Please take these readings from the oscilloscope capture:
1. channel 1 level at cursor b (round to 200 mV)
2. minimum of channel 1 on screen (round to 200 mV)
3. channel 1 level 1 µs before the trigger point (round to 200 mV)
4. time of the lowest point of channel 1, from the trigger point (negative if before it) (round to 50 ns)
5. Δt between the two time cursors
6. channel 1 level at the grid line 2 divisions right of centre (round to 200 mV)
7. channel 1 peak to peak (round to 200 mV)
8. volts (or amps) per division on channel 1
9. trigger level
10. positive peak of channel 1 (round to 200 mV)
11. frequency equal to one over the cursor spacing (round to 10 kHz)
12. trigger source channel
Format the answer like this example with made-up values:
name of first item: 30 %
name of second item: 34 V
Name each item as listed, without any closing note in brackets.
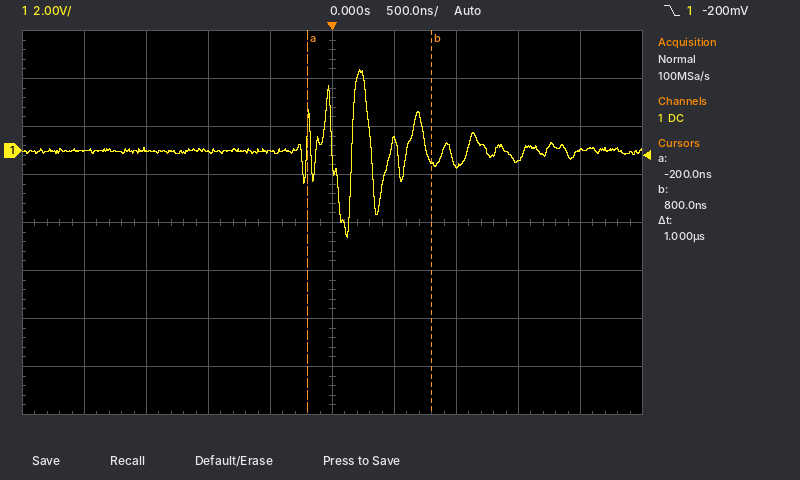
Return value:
channel 1 level at cursor b: -400 mV
minimum of channel 1 on screen: -3.6 V
channel 1 level 1 µs before the trigger point: 0.0 V
time of the lowest point of channel 1, from the trigger point (negative if before it): +100 ns
Δt between the two time cursors: 1 µs
channel 1 level at the grid line 2 divisions right of centre: -600 mV
channel 1 peak to peak: 7.0 V
volts (or amps) per division on channel 1: 2 V
trigger level: -200 mV
positive peak of channel 1: 3.4 V
frequency equal to one over the cursor spacing: 1.00 MHz
trigger source channel: channel 1
